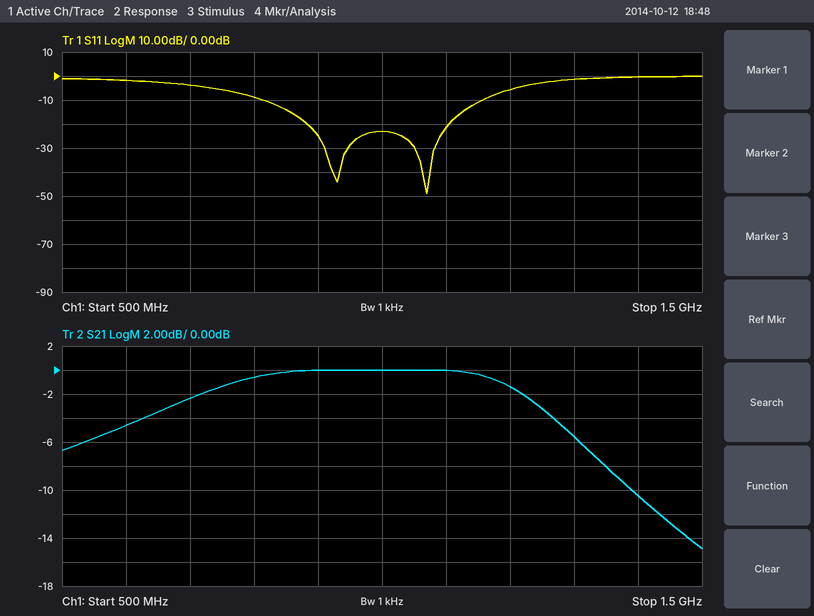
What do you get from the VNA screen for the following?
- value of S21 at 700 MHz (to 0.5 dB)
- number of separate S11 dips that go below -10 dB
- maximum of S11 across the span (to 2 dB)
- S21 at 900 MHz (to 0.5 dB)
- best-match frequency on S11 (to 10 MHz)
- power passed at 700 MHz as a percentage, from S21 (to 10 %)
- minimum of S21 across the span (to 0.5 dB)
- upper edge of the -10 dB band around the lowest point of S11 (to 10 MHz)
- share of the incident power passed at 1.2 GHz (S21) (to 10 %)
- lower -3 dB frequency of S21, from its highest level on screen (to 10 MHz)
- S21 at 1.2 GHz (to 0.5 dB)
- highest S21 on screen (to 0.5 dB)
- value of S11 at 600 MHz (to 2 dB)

-2.5 dB
2
0 dB
0.0 dB
1.07 GHz
60 %
-15.0 dB
1.16 GHz
70 %
670 MHz
-1.5 dB
0.0 dB
-2 dB
